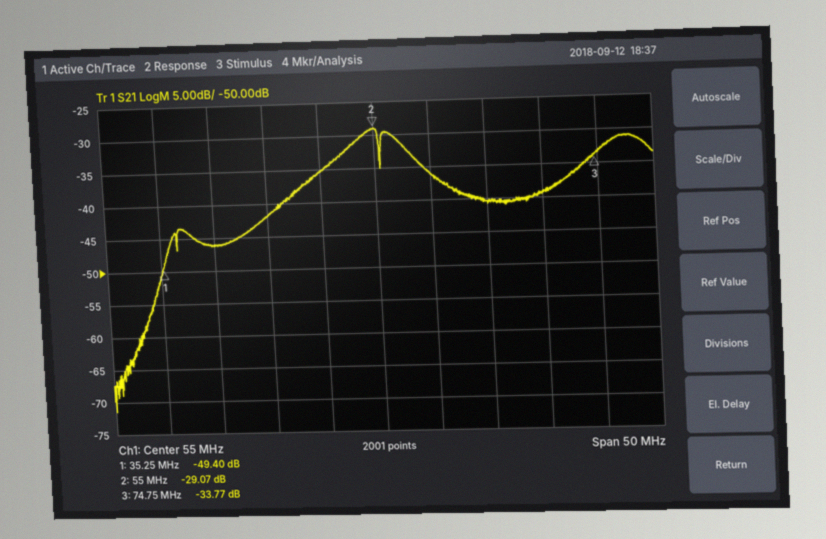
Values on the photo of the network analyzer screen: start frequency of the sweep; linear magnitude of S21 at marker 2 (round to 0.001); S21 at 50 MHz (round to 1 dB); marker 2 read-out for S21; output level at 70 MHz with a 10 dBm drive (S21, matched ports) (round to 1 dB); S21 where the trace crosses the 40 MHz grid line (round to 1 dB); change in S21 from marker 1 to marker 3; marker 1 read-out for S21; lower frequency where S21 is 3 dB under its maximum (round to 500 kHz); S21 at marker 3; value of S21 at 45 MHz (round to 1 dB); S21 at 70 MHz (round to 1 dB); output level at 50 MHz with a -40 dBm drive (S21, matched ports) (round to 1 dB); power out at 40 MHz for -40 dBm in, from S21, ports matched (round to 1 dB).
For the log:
30 MHz
0.035
-35 dB
-29.07 dB
-29 dBm
-46 dB
15.63 dB
-49.40 dB
52.5 MHz
-33.77 dB
-42 dB
-39 dB
-75 dBm
-86 dBm
